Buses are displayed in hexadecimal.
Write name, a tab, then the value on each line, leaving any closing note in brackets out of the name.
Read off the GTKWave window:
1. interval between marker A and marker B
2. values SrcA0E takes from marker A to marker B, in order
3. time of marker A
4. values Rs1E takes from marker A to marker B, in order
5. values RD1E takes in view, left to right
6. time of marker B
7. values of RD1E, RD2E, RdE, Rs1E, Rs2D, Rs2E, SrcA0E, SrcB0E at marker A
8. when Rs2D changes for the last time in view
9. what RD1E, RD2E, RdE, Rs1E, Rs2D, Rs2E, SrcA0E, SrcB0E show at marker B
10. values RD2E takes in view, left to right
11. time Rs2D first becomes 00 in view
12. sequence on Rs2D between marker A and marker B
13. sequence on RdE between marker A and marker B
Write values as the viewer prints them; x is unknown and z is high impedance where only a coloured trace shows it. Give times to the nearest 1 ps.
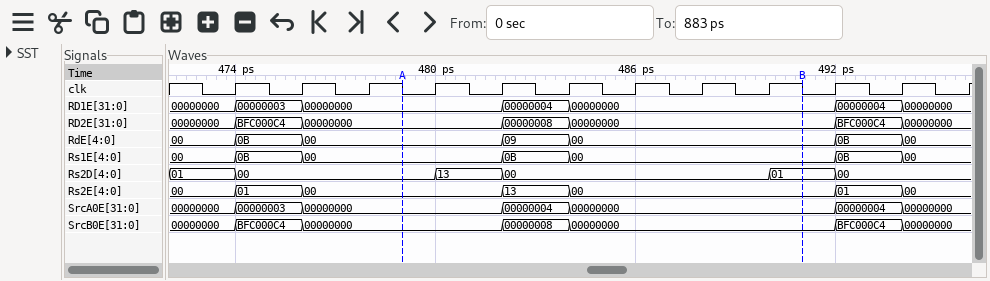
interval between marker A and marker B	12 ps
values SrcA0E takes from marker A to marker B, in order	00000000, 00000004, 00000000
time of marker A	479 ps
values Rs1E takes from marker A to marker B, in order	00, 0B, 00
values RD1E takes in view, left to right	00000000, 00000003, 00000000, 00000004, 00000000, 00000004, 00000000
time of marker B	491 ps
values of RD1E, RD2E, RdE, Rs1E, Rs2D, Rs2E, SrcA0E, SrcB0E at marker A	RD1E=00000000, RD2E=00000000, RdE=00, Rs1E=00, Rs2D=00, Rs2E=00, SrcA0E=00000000, SrcB0E=00000000
when Rs2D changes for the last time in view	492 ps
what RD1E, RD2E, RdE, Rs1E, Rs2D, Rs2E, SrcA0E, SrcB0E show at marker B	RD1E=00000000, RD2E=00000000, RdE=00, Rs1E=00, Rs2D=01, Rs2E=00, SrcA0E=00000000, SrcB0E=00000000
values RD2E takes in view, left to right	00000000, BFC000C4, 00000000, 00000008, 00000000, BFC000C4, 00000000
time Rs2D first becomes 00 in view	474 ps
sequence on Rs2D between marker A and marker B	00, 13, 00, 01
sequence on RdE between marker A and marker B	00, 09, 00
